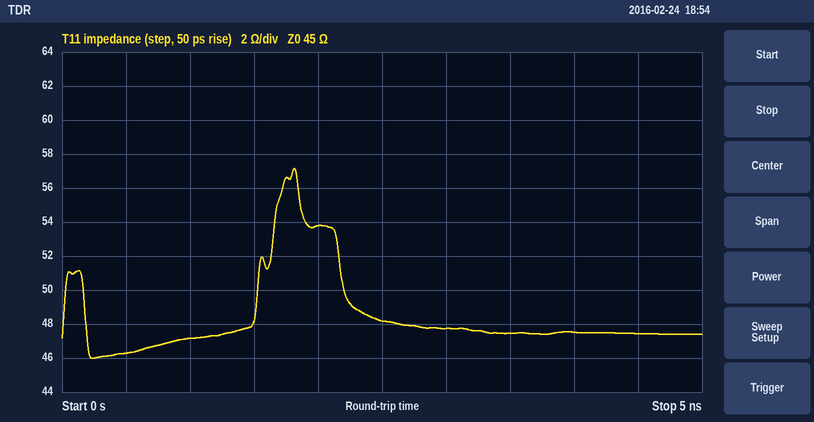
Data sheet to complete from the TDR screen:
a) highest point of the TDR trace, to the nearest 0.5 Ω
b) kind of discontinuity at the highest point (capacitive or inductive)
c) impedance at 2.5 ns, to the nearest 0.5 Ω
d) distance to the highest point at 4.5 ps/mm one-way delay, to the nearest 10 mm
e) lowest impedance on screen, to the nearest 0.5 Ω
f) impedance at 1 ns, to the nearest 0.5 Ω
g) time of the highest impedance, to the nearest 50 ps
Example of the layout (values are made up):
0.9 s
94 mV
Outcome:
57.0 Ω
inductive
48.0 Ω
200 mm
46.0 Ω
47.0 Ω
1.80 ns
